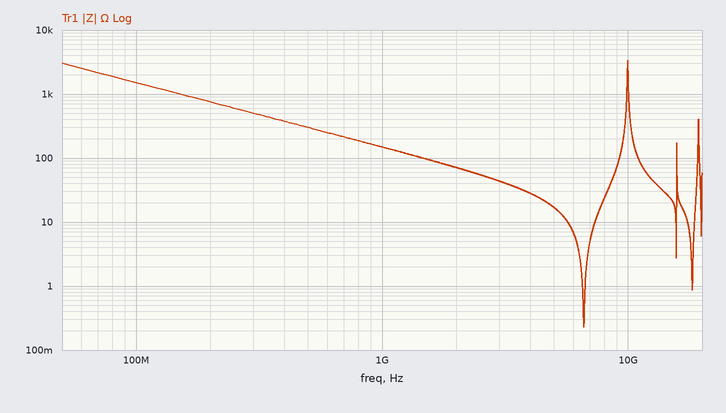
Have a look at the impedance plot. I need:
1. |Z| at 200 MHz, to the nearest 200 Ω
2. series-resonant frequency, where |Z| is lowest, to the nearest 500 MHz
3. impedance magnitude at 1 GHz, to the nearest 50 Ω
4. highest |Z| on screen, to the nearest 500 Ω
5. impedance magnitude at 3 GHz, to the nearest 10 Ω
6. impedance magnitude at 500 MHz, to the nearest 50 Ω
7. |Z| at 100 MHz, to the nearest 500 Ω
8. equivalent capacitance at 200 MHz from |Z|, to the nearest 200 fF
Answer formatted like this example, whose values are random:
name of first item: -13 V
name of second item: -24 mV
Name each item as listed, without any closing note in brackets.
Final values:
|Z| at 200 MHz, to the nearest 200 Ω: 800 Ω
series-resonant frequency, where |Z| is lowest, to the nearest 500 MHz: 6.5 GHz
impedance magnitude at 1 GHz, to the nearest 50 Ω: 150 Ω
highest |Z| on screen, to the nearest 500 Ω: 3.5 kΩ
impedance magnitude at 3 GHz, to the nearest 10 Ω: 40 Ω
impedance magnitude at 500 MHz, to the nearest 50 Ω: 300 Ω
|Z| at 100 MHz, to the nearest 500 Ω: 1.5 kΩ
equivalent capacitance at 200 MHz from |Z|, to the nearest 200 fF: 1.0 pF
